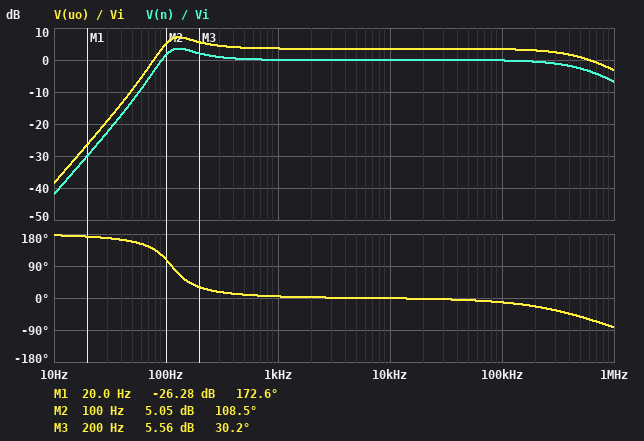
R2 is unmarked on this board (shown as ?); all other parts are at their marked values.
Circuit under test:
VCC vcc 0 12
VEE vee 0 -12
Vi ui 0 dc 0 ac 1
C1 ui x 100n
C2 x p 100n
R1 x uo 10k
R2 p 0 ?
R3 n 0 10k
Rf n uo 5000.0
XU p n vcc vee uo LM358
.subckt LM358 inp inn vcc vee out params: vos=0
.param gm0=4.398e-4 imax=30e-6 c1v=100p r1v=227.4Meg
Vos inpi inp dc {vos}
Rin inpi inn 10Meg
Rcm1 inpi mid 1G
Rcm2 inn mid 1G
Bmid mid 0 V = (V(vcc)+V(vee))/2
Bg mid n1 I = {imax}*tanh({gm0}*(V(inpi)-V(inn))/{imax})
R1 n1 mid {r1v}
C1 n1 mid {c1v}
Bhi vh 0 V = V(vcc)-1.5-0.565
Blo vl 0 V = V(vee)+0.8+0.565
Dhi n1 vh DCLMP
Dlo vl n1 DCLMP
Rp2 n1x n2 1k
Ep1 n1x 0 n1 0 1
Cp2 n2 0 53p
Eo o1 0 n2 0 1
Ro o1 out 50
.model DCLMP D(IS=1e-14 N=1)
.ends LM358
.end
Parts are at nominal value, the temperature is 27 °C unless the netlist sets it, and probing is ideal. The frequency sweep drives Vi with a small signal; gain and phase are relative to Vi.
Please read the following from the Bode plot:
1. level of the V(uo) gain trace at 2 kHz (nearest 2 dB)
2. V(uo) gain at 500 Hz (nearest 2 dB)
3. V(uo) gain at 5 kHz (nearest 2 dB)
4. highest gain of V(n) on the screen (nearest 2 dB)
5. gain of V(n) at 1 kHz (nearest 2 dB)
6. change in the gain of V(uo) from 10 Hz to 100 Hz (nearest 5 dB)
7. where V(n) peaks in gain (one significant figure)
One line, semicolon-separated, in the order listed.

4 dB; 4 dB; 4 dB; 4 dB; 0 dB; 45 dB; 100 Hz
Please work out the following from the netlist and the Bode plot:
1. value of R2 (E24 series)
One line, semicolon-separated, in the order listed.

20 kΩ
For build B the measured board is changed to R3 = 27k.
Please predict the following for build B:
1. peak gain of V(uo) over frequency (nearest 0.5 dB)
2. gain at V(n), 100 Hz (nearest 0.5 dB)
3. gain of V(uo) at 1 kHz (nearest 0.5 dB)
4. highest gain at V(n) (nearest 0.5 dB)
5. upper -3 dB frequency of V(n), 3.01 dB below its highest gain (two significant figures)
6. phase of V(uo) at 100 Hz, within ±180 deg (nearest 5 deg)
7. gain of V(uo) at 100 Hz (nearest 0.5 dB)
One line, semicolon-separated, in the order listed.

2.0 dB; -2.5 dB; 1.5 dB; 0.5 dB; 640 kHz; 100 deg; -1.0 dB
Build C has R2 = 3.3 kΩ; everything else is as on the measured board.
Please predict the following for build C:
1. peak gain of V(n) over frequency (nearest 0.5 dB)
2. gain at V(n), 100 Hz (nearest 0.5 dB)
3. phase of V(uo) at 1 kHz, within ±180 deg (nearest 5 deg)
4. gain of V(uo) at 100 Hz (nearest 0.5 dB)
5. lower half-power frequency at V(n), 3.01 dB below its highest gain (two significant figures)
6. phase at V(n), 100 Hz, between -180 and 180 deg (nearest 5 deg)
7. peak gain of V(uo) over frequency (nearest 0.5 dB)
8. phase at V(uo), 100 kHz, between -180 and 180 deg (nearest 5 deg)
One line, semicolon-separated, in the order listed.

0 dB; -21.0 dB; 45 deg; -17.5 dB; 800 Hz; 125 deg; 3.5 dB; -10 deg
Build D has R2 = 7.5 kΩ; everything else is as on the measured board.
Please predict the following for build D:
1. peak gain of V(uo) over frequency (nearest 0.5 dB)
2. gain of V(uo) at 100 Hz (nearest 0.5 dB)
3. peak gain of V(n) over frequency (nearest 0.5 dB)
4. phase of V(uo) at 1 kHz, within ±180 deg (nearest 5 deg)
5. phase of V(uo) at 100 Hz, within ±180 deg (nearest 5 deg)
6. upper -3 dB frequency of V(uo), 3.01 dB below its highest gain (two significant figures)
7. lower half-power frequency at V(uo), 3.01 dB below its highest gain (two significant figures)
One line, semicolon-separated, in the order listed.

3.5 dB; -9.0 dB; 0 dB; 20 deg; 125 deg; 540 kHz; 260 Hz
